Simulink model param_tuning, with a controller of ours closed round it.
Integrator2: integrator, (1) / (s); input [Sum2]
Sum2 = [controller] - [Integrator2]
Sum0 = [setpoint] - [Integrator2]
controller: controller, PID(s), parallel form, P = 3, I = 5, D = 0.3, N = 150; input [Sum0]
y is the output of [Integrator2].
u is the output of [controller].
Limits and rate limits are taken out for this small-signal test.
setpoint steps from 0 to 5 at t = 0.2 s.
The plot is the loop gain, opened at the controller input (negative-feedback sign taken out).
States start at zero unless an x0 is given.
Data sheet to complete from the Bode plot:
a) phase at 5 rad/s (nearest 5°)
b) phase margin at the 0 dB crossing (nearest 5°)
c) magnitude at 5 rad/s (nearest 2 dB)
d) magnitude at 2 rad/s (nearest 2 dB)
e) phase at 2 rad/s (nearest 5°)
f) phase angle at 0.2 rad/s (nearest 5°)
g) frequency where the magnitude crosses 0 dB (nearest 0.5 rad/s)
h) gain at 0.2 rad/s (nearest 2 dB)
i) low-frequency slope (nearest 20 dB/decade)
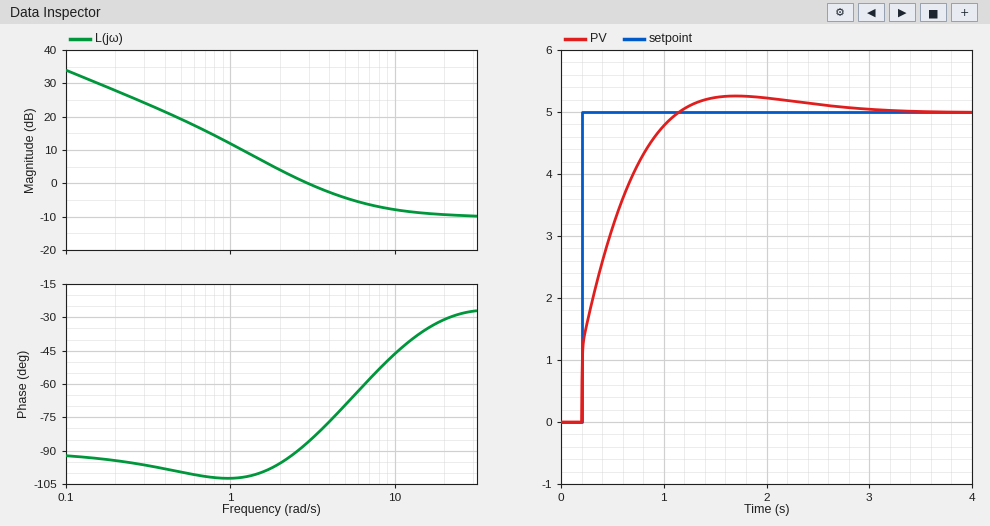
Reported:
-70°
95°
-4 dB
4 dB
-95°
-95°
3.0 rad/s
28 dB
-20 dB/decade
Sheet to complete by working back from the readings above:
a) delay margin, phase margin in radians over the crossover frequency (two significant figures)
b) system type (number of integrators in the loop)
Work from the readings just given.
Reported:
0.55 s
1
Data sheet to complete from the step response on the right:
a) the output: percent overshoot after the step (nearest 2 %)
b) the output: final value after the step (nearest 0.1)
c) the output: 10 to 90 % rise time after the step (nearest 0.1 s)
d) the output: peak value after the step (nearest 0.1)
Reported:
6 %
5.0
0.7 s
5.3
